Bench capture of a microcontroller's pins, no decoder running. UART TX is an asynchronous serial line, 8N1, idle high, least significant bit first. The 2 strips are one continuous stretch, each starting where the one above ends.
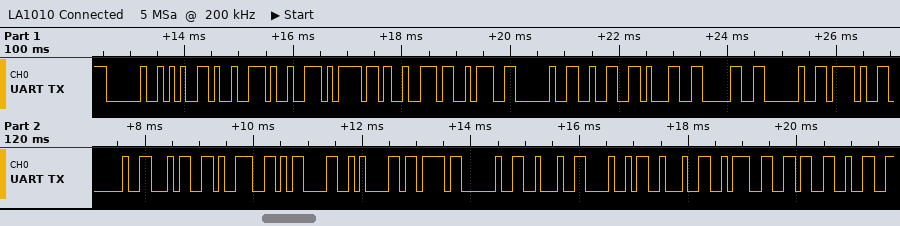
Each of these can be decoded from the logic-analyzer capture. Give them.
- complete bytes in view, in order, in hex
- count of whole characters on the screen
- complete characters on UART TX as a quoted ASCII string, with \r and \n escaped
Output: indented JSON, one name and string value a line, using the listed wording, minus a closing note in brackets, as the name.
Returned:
{
  "complete bytes in view, in order, in hex": "20 65 72 72 6F 72 3A 20 32 31 30 20 2F 20 34 39 0D 0A 7B 20 22 48 22 3A 36 32",
  "count of whole characters on the screen": "26",
  "complete characters on UART TX as a quoted ASCII string, with \\r and \\n escaped": "\" error: 210 / 49\\r\\n{ \\\"H\\\":62\""
}
